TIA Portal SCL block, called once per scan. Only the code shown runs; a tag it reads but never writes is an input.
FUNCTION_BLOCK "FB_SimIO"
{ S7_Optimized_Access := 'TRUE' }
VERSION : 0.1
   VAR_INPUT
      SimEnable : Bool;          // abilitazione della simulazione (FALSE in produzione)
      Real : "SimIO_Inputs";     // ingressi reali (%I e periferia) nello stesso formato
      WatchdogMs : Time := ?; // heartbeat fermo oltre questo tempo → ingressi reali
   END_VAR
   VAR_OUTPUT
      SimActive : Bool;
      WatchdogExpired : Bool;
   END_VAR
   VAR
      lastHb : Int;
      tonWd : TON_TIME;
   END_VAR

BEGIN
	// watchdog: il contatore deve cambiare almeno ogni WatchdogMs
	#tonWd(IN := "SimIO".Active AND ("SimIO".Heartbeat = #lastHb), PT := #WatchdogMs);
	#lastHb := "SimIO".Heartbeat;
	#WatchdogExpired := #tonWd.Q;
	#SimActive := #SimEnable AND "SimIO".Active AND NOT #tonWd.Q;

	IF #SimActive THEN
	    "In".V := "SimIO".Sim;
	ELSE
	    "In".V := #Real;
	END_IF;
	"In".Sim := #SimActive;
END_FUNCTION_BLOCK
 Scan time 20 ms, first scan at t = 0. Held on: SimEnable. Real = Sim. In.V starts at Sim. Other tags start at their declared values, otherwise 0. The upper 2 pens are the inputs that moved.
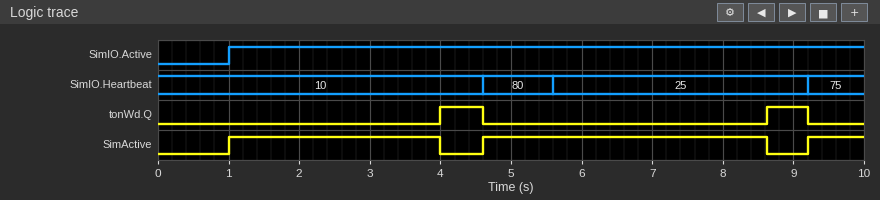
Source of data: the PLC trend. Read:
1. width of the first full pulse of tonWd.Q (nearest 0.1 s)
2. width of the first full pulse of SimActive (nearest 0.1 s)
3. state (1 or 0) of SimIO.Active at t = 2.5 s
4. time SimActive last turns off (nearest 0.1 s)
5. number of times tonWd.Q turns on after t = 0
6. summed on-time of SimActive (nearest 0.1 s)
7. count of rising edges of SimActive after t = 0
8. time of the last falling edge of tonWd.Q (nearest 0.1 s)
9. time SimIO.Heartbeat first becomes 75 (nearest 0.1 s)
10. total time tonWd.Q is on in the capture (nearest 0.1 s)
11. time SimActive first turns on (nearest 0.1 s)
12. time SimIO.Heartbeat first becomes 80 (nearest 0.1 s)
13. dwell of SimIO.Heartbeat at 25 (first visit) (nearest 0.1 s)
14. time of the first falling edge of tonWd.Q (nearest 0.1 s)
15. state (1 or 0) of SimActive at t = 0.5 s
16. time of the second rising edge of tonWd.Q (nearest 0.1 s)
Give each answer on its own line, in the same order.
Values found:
0.6 s
3.0 s
1
8.6 s
2
7.8 s
3
9.2 s
9.2 s
1.2 s
1.0 s
4.6 s
3.6 s
4.6 s
0
8.6 s
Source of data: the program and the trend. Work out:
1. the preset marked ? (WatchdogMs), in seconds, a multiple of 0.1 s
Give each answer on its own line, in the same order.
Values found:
3.0 s
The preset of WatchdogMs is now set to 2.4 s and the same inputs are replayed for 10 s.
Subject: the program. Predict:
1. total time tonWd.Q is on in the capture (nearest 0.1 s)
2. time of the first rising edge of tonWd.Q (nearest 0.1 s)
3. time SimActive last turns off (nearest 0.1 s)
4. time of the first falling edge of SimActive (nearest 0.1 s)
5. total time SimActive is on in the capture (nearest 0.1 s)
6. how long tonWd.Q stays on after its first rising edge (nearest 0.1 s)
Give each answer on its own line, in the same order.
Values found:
2.4 s
3.4 s
8.0 s
3.4 s
6.6 s
1.2 s
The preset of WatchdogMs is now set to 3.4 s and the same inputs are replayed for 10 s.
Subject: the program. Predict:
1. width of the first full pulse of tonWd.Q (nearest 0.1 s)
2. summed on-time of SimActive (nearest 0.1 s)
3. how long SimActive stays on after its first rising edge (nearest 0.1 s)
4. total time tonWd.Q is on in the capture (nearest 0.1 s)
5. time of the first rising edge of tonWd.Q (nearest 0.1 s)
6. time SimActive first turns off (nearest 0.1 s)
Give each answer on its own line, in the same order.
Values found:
0.2 s
8.6 s
3.4 s
0.4 s
4.4 s
4.4 s
